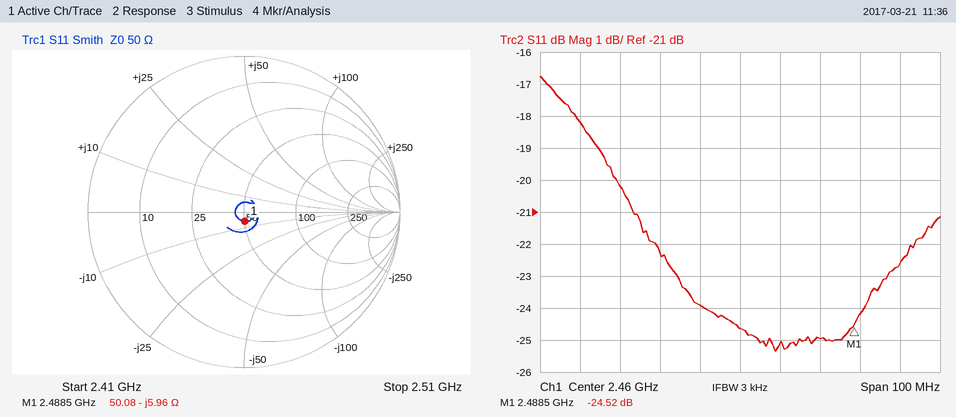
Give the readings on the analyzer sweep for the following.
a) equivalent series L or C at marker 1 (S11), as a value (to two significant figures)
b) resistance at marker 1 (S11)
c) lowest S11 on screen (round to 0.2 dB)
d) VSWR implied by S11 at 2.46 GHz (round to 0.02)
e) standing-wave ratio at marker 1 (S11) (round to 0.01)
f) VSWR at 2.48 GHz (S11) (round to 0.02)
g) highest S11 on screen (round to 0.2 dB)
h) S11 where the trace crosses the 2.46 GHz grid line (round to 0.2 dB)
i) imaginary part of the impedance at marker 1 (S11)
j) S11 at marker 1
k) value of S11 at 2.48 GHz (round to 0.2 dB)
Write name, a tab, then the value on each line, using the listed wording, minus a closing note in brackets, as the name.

equivalent series L or C at marker 1 (S11), as a value	11 pF
resistance at marker 1	50.08 Ω
lowest S11 on screen	-25.4 dB
VSWR implied by S11 at 2.46 GHz	1.12
standing-wave ratio at marker 1 (S11)	1.13
VSWR at 2.48 GHz (S11)	1.12
highest S11 on screen	-16.8 dB
S11 where the trace crosses the 2.46 GHz grid line	-24.6 dB
imaginary part of the impedance at marker 1	-5.96 Ω
S11 at marker 1	-24.52 dB
value of S11 at 2.48 GHz	-25.0 dB
